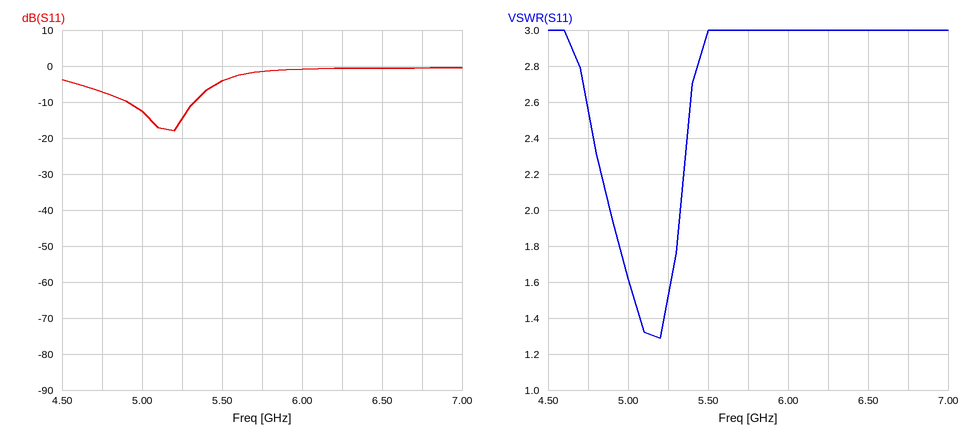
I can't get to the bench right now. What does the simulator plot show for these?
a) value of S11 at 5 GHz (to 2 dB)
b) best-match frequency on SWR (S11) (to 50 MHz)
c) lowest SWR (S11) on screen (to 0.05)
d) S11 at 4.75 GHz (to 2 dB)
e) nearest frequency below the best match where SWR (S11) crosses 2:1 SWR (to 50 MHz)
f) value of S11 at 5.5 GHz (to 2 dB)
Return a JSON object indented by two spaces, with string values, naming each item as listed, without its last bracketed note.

{
  "value of S11 at 5 GHz": "-12 dB",
  "best-match frequency on SWR (S11)": "5.20 GHz",
  "lowest SWR (S11) on screen": "1.30",
  "S11 at 4.75 GHz": "-8 dB",
  "nearest frequency below the best match where SWR (S11) crosses 2:1 SWR": "4.90 GHz",
  "value of S11 at 5.5 GHz": "-4 dB"
}
